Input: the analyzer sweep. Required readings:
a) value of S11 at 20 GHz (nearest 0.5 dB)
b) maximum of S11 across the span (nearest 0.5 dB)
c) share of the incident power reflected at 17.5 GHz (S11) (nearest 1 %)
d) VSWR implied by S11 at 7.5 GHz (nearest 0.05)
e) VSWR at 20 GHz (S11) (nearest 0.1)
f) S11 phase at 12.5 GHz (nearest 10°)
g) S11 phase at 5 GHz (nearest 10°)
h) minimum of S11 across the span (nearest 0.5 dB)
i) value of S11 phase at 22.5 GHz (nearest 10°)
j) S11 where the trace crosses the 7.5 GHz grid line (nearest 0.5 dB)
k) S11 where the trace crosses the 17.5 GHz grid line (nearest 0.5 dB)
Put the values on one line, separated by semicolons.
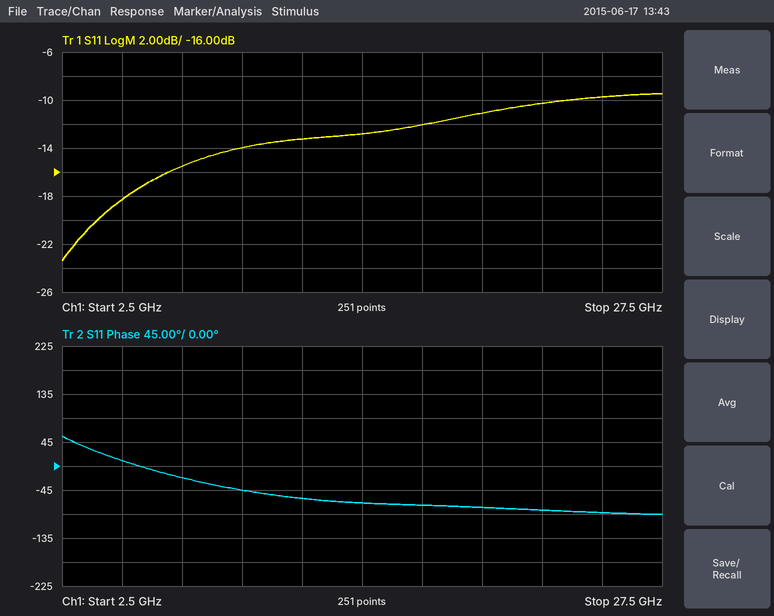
-11.0 dB; -9.5 dB; 6 %; 1.40; 1.8; -60°; 10°; -23.5 dB; -80°; -15.5 dB; -12.0 dB
